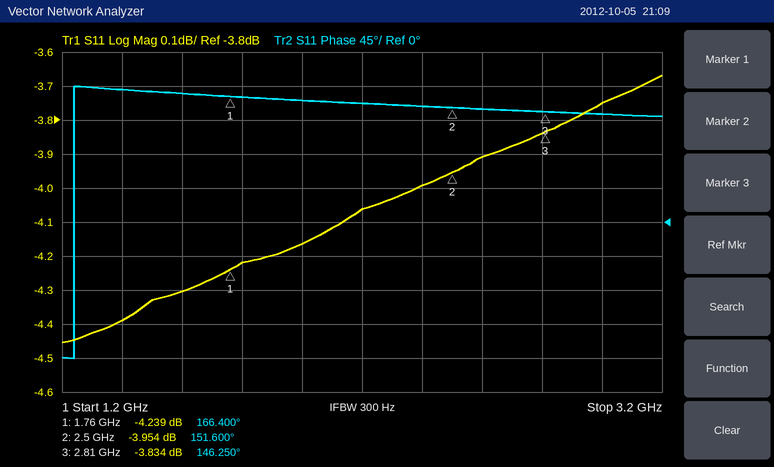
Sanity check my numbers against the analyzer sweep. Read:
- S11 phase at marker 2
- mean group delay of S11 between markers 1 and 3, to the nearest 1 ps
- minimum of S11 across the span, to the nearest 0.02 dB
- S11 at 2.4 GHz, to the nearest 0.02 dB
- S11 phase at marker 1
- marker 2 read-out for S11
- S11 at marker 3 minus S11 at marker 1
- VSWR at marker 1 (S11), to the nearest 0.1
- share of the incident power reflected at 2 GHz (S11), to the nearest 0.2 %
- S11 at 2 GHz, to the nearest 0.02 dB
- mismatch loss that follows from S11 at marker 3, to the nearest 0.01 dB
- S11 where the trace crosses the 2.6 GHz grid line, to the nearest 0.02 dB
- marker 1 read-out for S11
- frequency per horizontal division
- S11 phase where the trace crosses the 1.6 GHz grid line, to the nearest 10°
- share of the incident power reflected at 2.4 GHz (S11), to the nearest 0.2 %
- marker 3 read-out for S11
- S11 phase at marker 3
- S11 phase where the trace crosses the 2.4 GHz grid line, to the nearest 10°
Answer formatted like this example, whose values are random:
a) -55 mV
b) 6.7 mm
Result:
a) 151.600°
b) 53 ps
c) -4.46 dB
d) -4.00 dB
e) 166.400°
f) -3.954 dB
g) 0.405 dB
h) 4.2
i) 38.4 %
j) -4.16 dB
k) 2.32 dB
l) -3.90 dB
m) -4.239 dB
n) 200 MHz
o) 170°
p) 39.8 %
q) -3.834 dB
r) 146.250°
s) 150°
